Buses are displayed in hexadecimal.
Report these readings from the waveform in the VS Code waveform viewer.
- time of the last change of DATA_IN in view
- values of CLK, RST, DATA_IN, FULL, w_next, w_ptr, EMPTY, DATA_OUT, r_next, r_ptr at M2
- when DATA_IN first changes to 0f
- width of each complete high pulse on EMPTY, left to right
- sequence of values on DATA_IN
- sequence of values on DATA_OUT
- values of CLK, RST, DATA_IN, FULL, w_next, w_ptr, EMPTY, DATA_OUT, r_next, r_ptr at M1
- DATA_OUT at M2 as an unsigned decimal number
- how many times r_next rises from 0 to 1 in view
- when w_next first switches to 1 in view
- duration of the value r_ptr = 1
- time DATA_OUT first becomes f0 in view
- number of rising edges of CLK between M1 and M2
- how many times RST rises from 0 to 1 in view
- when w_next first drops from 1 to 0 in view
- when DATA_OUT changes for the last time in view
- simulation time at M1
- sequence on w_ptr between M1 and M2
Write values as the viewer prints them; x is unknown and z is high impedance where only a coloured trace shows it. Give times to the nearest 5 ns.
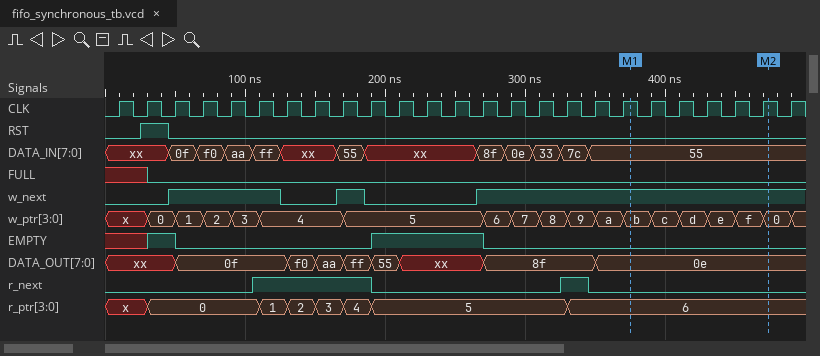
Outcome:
345 ns
CLK=1, RST=0, DATA_IN=55, FULL=0, w_next=1, w_ptr=0, EMPTY=0, DATA_OUT=0e, r_next=0, r_ptr=6
45 ns
80 ns
xx, 0f, f0, aa, ff, xx, 55, xx, 8f, 0e, 33, 7c, 55
xx, 0f, f0, aa, ff, 55, xx, 8f, 0e
CLK=1, RST=0, DATA_IN=55, FULL=0, w_next=1, w_ptr=b, EMPTY=0, DATA_OUT=0e, r_next=0, r_ptr=6
14
2
45 ns
20 ns
130 ns
5
1
125 ns
350 ns
375 ns
b, c, d, e, f, 0
